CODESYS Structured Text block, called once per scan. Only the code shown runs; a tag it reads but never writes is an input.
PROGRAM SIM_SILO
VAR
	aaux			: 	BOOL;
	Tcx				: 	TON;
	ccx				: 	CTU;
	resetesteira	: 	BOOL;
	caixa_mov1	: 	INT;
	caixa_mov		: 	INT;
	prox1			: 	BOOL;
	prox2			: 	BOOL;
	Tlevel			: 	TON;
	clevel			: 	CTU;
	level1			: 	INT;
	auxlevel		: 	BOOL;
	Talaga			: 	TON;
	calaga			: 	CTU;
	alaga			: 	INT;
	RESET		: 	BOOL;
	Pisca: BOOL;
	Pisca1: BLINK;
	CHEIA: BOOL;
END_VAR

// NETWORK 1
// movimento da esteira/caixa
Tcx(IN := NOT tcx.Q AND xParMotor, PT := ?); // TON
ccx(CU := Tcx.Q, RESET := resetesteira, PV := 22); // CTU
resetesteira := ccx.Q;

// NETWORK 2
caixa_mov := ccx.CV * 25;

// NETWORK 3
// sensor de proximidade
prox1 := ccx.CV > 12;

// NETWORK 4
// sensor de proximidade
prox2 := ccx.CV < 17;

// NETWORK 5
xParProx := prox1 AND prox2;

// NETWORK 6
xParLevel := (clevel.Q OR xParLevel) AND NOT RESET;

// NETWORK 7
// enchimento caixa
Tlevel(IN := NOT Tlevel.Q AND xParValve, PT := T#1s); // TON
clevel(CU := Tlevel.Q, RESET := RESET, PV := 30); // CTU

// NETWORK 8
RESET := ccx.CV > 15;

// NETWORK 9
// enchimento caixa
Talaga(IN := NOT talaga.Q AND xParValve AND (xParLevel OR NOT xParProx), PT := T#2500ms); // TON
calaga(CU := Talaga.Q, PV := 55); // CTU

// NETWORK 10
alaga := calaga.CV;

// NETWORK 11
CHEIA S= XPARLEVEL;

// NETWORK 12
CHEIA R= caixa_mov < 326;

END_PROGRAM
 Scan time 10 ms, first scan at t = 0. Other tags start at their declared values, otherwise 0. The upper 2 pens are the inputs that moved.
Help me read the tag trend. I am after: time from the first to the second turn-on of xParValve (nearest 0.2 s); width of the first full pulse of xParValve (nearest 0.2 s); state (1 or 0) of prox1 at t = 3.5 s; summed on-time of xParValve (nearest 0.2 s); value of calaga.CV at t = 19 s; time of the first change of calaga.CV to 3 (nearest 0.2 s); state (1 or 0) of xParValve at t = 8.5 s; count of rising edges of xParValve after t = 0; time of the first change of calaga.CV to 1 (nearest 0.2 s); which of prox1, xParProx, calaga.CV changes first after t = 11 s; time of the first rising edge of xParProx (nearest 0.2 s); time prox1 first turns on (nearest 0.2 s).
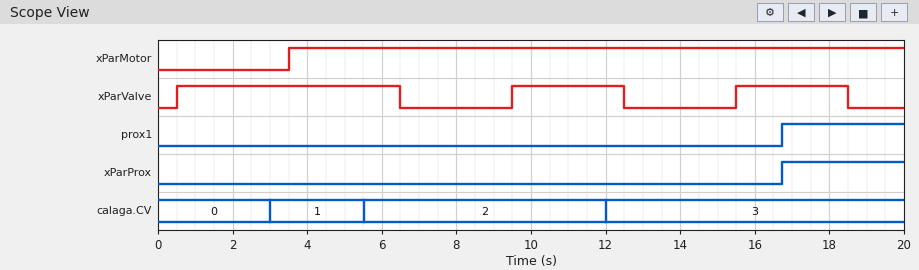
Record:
9.0 s
6.0 s
0
12.0 s
3
12.0 s
0
3
3.0 s
calaga.CV
16.8 s
16.8 s
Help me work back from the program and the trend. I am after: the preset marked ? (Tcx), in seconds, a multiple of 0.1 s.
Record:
1.0 s
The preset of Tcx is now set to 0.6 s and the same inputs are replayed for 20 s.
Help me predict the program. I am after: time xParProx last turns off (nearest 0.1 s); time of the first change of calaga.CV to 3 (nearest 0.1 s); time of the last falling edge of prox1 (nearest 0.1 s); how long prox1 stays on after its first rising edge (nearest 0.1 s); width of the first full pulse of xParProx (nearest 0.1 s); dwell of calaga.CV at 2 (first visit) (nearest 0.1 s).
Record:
14.0 s
18.0 s
17.1 s
5.6 s
2.5 s
12.5 s
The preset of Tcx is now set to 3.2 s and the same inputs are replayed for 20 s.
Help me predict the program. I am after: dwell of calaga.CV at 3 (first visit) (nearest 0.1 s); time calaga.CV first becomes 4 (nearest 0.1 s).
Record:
6.0 s
18.0 s
